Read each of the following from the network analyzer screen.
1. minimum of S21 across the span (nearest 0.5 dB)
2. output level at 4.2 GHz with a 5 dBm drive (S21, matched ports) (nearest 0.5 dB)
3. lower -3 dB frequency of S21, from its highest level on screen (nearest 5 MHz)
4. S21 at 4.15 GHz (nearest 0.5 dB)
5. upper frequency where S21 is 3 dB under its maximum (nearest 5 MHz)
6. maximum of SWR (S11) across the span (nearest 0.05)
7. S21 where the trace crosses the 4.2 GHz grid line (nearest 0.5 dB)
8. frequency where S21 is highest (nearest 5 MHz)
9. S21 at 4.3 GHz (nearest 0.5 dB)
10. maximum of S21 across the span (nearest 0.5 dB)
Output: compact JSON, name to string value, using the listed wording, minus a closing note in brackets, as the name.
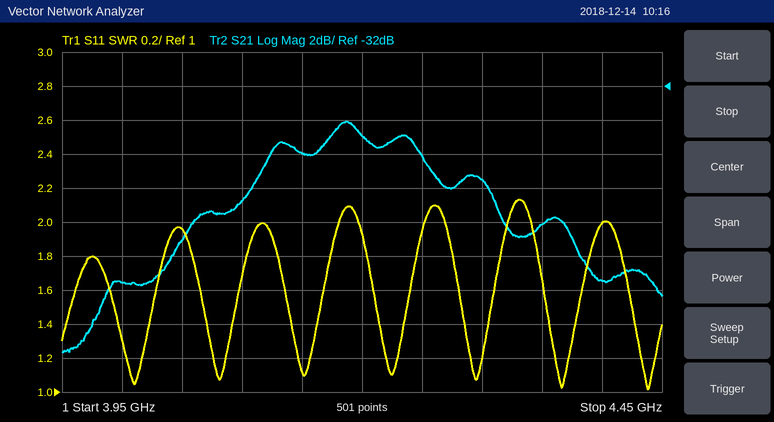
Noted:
{"minimum of S21 across the span": "-47.5 dB", "output level at 4.2 GHz with a 5 dBm drive (S21, matched ports)": "-30.0 dBm", "lower -3 dB frequency of S21, from its highest level on screen": "4.115 GHz", "S21 at 4.15 GHz": "-36.0 dB", "upper frequency where S21 is 3 dB under its maximum": "4.260 GHz", "maximum of SWR (S11) across the span": "2.15", "S21 where the trace crosses the 4.2 GHz grid line": "-35.0 dB", "frequency where S21 is highest": "4.185 GHz", "S21 at 4.3 GHz": "-37.5 dB", "maximum of S21 across the span": "-34.0 dB"}
